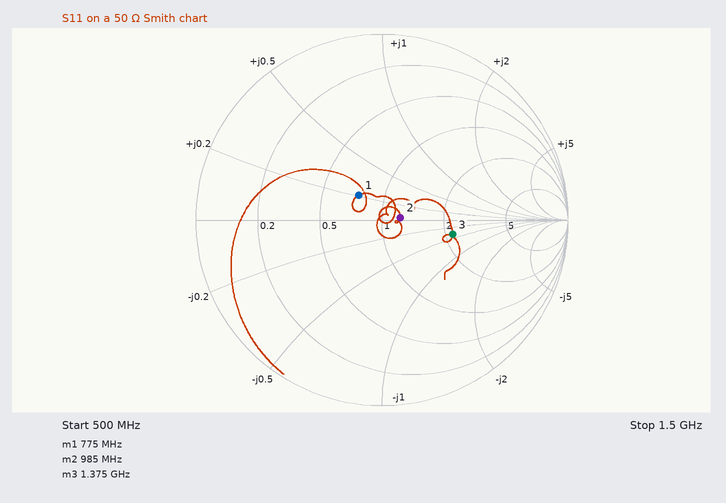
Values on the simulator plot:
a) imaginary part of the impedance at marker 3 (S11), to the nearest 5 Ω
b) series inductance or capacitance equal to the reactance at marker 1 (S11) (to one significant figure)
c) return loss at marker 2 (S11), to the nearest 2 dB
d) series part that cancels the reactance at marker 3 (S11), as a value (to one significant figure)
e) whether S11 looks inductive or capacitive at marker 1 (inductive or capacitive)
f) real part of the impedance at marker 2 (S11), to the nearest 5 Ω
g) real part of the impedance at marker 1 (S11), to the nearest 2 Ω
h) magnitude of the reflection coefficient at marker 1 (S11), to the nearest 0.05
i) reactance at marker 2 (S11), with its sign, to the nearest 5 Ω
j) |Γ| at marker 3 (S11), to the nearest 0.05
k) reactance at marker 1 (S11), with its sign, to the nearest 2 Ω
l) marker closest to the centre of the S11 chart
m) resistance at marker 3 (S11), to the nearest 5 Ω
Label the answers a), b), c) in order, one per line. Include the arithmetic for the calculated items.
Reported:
a) -20 Ω
b) L = 10 Ω/(2π × 775 MHz) ≈ 2 nH
c) 20 dB
d) L = 20 Ω/(2π × 1.375 GHz) ≈ 2 nH
e) inductive
f) 60 Ω
g) 38 Ω
h) 0.20
i) 0 Ω
j) 0.40
k) +10 Ω
l) marker 2
m) 110 Ω
